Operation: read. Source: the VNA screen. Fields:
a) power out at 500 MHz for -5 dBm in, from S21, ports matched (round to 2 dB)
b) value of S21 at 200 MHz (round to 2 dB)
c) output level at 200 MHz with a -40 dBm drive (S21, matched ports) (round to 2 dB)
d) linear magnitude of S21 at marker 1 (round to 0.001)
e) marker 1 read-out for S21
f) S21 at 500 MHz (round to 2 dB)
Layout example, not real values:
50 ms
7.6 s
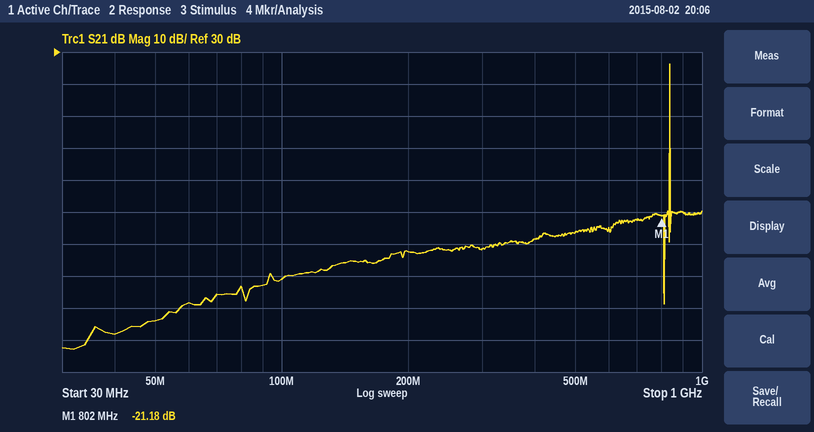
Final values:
-32 dBm
-32 dB
-72 dBm
0.087
-21.18 dB
-26 dB
